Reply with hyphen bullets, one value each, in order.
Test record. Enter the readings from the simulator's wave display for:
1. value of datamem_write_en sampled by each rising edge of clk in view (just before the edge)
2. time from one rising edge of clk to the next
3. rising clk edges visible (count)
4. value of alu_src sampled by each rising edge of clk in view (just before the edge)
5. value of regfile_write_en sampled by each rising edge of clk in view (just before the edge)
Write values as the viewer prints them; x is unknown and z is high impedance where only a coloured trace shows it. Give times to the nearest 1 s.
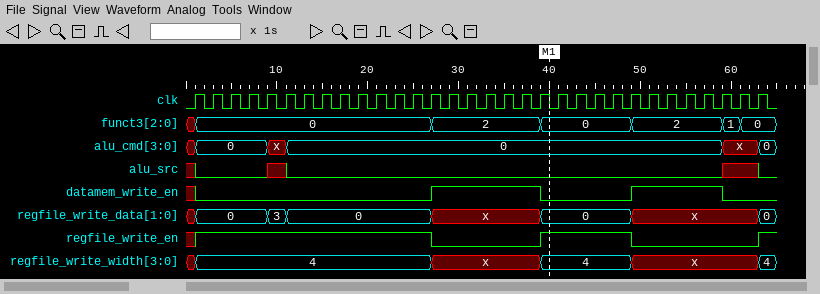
- x 0 0 0 0 0 0 0 0 0 0 0 0 0 1 1 1 1 1 1 0 0 0 0 0 1 1 1 1 1 0 0
- 2 s
- 32
- x 0 0 0 0 x 0 0 0 0 0 0 0 0 0 0 0 0 0 0 0 0 0 0 0 0 0 0 0 0 x x
- x 1 1 1 1 1 1 1 1 1 1 1 1 1 0 0 0 0 0 0 1 1 1 1 1 0 0 0 0 0 0 0
